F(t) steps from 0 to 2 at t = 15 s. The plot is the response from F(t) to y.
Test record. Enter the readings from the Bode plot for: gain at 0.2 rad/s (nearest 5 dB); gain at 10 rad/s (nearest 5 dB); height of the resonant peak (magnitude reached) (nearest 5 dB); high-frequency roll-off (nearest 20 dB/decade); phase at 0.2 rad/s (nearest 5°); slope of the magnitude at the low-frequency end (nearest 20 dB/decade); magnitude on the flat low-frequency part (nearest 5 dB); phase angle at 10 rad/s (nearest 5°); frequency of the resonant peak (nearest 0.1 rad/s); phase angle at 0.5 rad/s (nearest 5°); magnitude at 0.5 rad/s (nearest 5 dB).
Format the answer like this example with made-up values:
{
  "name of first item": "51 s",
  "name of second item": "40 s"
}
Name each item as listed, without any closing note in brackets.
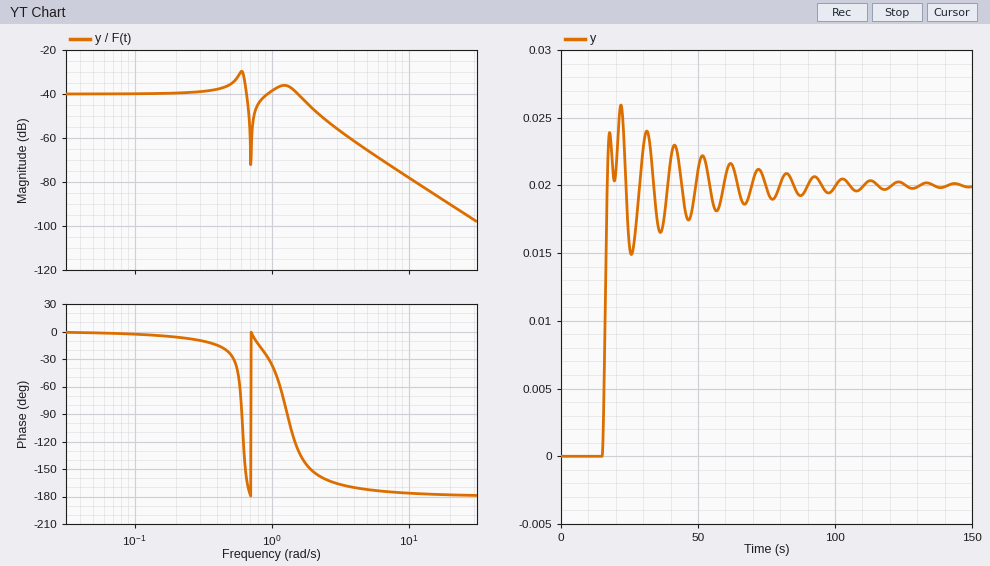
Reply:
{
  "gain at 0.2 rad/s": "-40 dB",
  "gain at 10 rad/s": "-80 dB",
  "height of the resonant peak (magnitude reached)": "-30 dB",
  "high-frequency roll-off": "-40 dB/decade",
  "phase at 0.2 rad/s": "-5°",
  "slope of the magnitude at the low-frequency end": "0 dB/decade",
  "magnitude on the flat low-frequency part": "-40 dB",
  "phase angle at 10 rad/s": "-175°",
  "frequency of the resonant peak": "0.6 rad/s",
  "phase angle at 0.5 rad/s": "-25°",
  "magnitude at 0.5 rad/s": "-35 dB"
}
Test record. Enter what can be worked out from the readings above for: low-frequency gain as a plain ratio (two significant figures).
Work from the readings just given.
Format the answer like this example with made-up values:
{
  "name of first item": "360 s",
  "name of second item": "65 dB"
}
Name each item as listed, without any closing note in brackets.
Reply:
{
  "low-frequency gain as a plain ratio": "0.010"
}
